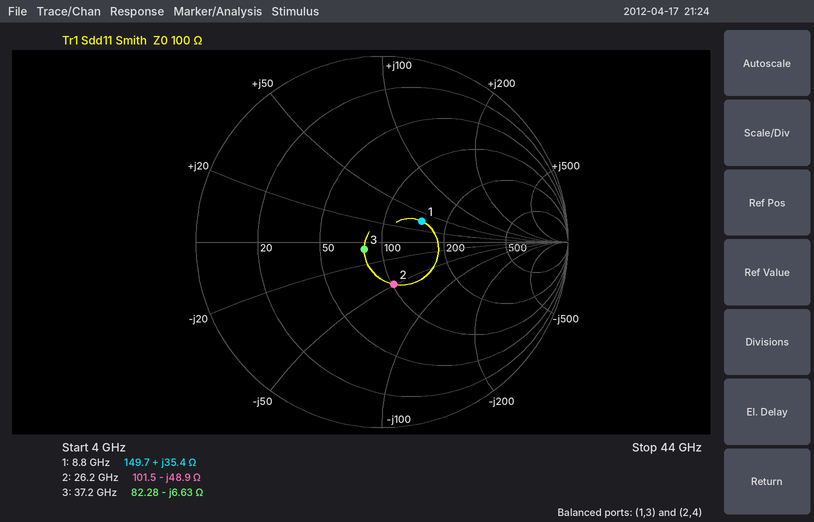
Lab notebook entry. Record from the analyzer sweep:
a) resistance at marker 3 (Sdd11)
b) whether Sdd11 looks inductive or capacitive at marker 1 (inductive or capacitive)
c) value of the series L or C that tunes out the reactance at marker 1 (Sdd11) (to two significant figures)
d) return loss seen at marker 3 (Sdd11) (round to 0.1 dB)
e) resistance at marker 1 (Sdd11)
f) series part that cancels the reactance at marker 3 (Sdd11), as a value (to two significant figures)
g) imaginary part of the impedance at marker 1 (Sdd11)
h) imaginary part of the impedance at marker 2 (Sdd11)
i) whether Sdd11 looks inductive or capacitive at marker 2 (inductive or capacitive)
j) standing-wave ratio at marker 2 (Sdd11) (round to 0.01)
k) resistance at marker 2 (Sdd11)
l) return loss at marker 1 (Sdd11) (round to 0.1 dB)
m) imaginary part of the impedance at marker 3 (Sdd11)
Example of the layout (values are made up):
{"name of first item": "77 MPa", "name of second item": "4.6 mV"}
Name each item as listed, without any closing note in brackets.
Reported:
{"resistance at marker 3": "82.28 Ω", "whether Sdd11 looks inductive or capacitive at marker 1": "inductive", "value of the series L or C that tunes out the reactance at marker 1 (Sdd11)": "510 fF", "return loss seen at marker 3 (Sdd11)": "19.7 dB", "resistance at marker 1": "149.7 Ω", "series part that cancels the reactance at marker 3 (Sdd11), as a value": "28 pH", "imaginary part of the impedance at marker 1": "+35.4 Ω", "imaginary part of the impedance at marker 2": "-48.9 Ω", "whether Sdd11 looks inductive or capacitive at marker 2": "capacitive", "standing-wave ratio at marker 2 (Sdd11)": "1.62", "resistance at marker 2": "101.5 Ω", "return loss at marker 1 (Sdd11)": "12.3 dB", "imaginary part of the impedance at marker 3": "-6.63 Ω"}
